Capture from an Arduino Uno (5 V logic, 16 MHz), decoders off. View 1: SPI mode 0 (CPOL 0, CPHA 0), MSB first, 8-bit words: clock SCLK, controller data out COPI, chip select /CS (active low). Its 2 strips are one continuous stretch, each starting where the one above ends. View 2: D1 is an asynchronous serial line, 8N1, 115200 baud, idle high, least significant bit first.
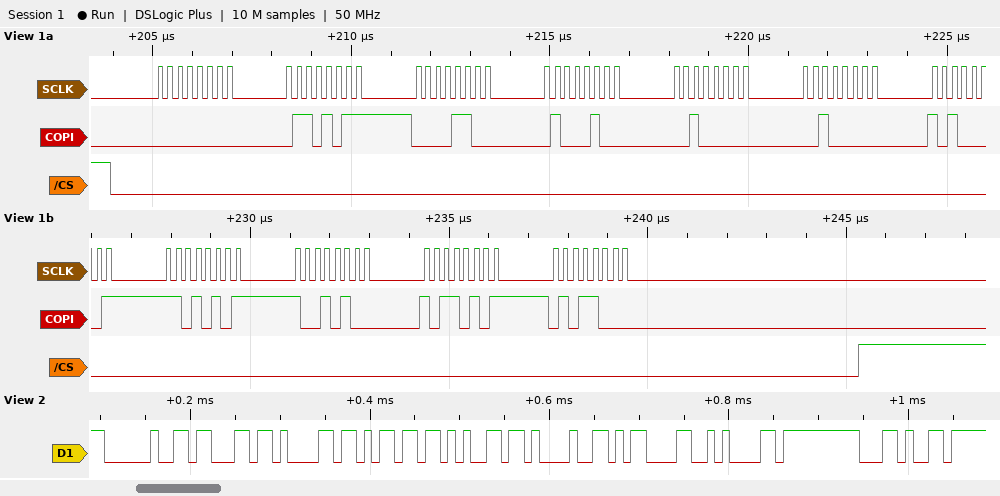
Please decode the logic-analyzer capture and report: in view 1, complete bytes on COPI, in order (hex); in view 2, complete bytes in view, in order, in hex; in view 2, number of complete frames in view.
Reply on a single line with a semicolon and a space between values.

00 6B 0C 44 20 20 A1 D5 94 B5 58; 20 63 61 6D 65 21 0D 0A FF 2C; 10
